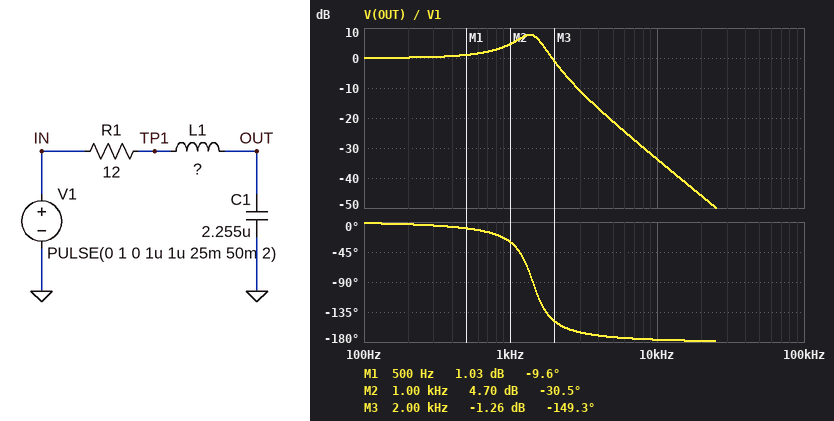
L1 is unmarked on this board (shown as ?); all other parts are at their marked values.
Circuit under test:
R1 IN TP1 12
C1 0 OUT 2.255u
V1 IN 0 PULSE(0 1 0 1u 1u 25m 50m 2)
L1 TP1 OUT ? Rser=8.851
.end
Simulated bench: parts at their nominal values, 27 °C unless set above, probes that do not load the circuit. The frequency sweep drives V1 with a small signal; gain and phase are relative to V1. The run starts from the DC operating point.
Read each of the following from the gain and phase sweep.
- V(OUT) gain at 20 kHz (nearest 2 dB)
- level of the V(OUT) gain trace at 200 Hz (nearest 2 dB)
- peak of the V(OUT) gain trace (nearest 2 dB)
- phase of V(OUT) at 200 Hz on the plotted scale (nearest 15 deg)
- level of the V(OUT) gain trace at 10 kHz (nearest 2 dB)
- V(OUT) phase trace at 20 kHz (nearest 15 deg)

-46 dB
0 dB
8 dB
0 deg
-34 dB
-180 deg
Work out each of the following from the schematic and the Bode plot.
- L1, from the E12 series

5.6 mH
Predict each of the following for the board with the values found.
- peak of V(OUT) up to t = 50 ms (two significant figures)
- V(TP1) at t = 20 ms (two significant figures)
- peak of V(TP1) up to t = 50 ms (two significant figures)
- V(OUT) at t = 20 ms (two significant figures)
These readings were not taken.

1.5 V
1.0 V
1.1 V
1.0 V
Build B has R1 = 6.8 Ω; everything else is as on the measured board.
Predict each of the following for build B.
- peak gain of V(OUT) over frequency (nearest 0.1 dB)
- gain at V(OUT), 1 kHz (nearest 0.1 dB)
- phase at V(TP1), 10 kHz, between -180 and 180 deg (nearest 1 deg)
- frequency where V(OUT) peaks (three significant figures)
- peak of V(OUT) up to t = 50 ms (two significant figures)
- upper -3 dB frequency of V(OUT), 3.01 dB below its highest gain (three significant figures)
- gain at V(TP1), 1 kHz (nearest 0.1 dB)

10.2 dB
5.2 dB
1 deg
1.38 kHz
1.6 V
1.59 kHz
-0.5 dB
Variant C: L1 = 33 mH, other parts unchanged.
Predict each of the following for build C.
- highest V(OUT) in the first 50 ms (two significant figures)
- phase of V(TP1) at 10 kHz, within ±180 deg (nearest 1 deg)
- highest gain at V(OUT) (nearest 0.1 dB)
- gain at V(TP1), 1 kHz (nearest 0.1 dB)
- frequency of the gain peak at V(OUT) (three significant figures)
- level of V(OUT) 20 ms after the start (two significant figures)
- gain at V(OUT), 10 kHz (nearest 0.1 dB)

1.8 V
0 deg
15.3 dB
-0.1 dB
579 Hz
1.0 V
-49.3 dB
